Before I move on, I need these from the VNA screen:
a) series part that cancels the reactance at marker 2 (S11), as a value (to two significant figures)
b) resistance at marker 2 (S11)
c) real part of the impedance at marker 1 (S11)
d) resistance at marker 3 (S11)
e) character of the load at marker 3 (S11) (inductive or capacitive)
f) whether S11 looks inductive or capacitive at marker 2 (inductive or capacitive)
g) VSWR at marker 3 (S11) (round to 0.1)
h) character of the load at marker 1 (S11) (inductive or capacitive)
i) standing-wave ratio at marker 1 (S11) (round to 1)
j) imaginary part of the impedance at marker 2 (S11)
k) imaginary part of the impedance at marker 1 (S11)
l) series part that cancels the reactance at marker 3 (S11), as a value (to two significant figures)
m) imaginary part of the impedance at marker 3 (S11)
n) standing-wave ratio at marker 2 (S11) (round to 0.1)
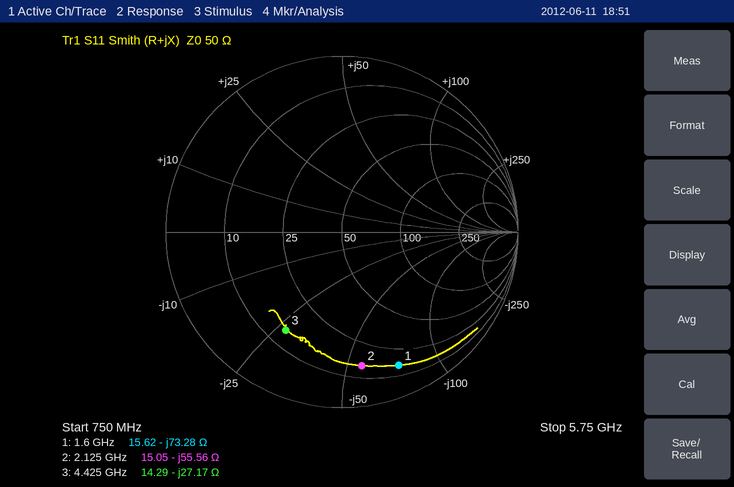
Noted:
4.2 nH
15.05 Ω
15.62 Ω
14.29 Ω
capacitive
capacitive
4.6
capacitive
10
-55.56 Ω
-73.28 Ω
980 pH
-27.17 Ω
7.6
